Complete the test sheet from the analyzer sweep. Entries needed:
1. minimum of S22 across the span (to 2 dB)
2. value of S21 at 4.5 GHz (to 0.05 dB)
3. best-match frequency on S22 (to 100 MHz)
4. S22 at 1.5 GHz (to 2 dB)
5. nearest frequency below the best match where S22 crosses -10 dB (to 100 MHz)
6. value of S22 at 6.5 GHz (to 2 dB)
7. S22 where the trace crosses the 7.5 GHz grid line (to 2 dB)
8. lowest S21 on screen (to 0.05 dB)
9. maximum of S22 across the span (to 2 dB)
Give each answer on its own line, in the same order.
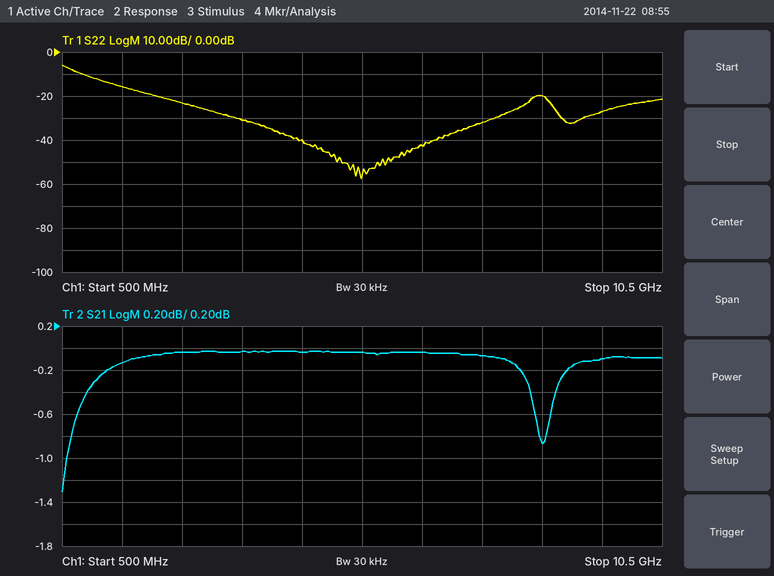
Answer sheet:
-58 dB
-0.05 dB
5.5 GHz
-16 dB
800 MHz
-42 dB
-32 dB
-1.30 dB
-6 dB
